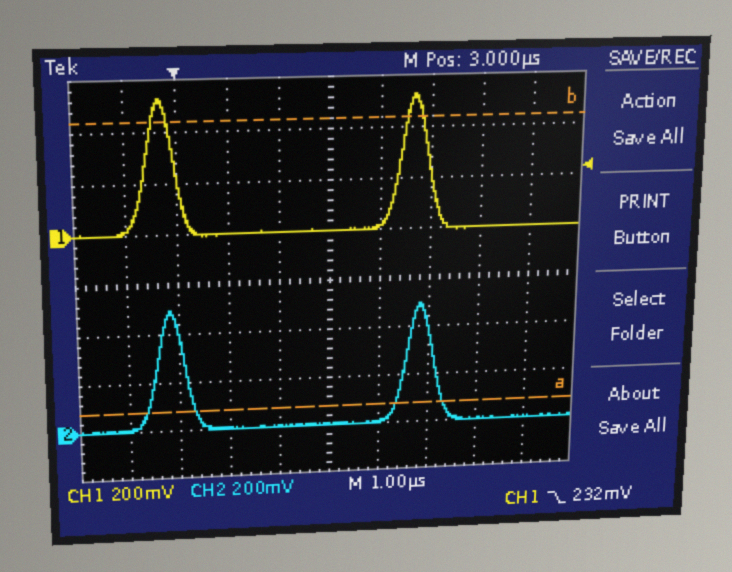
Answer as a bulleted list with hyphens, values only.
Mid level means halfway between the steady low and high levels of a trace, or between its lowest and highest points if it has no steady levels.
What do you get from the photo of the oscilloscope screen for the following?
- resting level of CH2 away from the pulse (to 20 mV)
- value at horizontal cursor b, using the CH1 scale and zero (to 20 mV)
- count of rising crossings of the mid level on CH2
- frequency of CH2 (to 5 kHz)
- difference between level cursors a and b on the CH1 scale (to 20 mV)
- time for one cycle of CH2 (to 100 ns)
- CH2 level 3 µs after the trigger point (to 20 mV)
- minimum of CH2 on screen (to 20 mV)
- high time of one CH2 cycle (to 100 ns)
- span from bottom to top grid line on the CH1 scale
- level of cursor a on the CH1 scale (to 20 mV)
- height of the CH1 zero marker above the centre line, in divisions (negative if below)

- 0 mV
- 440 mV
- 2
- 200 kHz
- 1.16 V
- 5.0 µs
- 0 mV
- 0 mV
- 600 ns
- 1.6 V
- -720 mV
- +1.0 div
